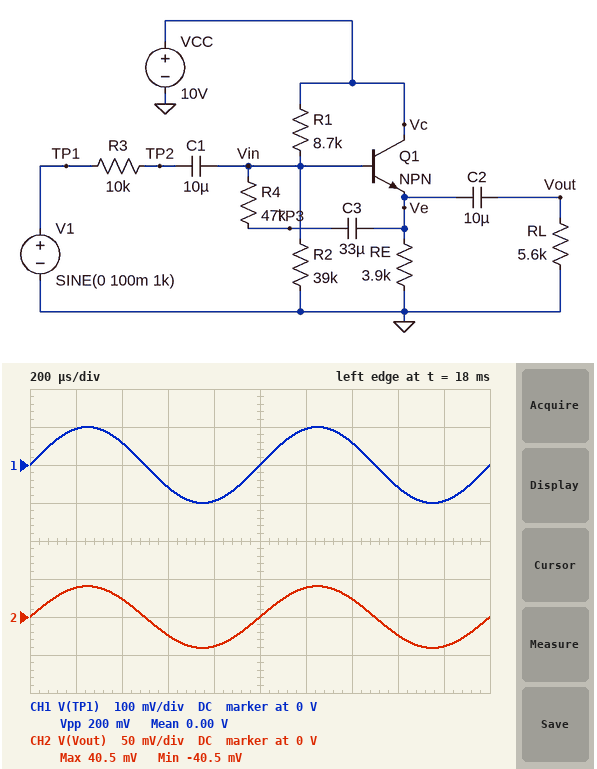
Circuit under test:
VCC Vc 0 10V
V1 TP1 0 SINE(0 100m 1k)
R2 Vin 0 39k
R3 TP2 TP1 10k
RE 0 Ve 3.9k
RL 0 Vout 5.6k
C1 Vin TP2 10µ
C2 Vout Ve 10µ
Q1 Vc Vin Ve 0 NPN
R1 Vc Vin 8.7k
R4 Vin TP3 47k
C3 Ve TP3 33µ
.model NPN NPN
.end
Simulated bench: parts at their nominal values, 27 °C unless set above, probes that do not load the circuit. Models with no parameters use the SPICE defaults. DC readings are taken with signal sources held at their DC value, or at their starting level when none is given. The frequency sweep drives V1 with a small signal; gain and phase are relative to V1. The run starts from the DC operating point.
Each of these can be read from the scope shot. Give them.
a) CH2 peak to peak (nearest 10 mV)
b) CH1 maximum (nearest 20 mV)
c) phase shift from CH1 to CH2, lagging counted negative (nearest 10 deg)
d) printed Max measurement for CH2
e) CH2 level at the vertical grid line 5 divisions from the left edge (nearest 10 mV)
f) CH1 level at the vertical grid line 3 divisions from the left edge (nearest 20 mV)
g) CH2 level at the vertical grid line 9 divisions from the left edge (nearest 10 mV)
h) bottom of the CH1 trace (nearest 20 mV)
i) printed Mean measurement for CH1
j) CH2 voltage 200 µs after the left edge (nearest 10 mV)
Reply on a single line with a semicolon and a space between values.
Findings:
80 mV; 100 mV; 0 deg; 40.5 mV; 0 V; -60 mV; -40 mV; -100 mV; 0.00 V; 40 mV
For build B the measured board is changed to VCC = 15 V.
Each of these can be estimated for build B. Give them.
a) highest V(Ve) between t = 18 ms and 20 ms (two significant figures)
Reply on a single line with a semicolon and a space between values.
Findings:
11 V
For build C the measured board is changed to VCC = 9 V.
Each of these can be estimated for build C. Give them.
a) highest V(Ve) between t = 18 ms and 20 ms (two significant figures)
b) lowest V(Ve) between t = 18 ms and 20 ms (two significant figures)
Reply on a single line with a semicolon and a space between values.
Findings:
6.5 V; 6.4 V
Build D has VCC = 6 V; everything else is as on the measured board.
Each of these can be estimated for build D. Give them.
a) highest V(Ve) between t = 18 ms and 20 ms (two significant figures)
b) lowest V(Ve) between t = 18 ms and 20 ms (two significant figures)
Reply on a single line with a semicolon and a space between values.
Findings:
4.1 V; 4.0 V
